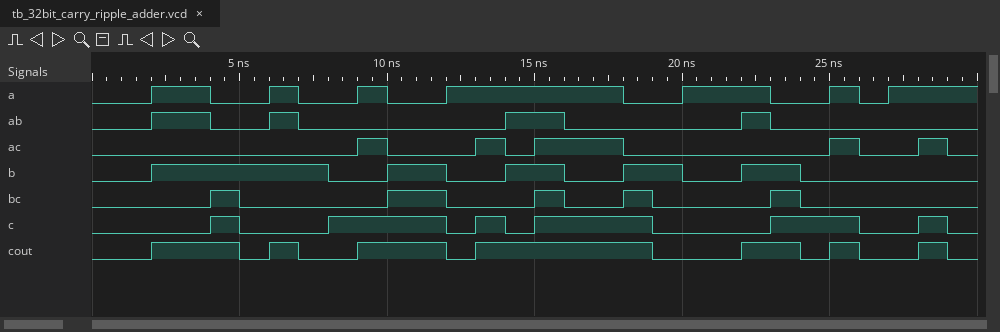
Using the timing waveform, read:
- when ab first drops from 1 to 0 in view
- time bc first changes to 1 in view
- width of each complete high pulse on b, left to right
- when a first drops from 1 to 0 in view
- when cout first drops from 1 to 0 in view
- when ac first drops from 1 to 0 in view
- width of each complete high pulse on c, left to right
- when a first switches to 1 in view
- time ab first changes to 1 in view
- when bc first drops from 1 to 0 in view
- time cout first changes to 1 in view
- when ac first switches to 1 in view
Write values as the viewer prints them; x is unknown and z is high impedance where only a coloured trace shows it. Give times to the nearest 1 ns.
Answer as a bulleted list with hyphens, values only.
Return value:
- 4 ns
- 4 ns
- 6 ns, 2 ns, 2 ns, 2 ns, 2 ns
- 4 ns
- 5 ns
- 10 ns
- 1 ns, 4 ns, 1 ns, 4 ns, 3 ns, 1 ns
- 2 ns
- 2 ns
- 5 ns
- 2 ns
- 9 ns
